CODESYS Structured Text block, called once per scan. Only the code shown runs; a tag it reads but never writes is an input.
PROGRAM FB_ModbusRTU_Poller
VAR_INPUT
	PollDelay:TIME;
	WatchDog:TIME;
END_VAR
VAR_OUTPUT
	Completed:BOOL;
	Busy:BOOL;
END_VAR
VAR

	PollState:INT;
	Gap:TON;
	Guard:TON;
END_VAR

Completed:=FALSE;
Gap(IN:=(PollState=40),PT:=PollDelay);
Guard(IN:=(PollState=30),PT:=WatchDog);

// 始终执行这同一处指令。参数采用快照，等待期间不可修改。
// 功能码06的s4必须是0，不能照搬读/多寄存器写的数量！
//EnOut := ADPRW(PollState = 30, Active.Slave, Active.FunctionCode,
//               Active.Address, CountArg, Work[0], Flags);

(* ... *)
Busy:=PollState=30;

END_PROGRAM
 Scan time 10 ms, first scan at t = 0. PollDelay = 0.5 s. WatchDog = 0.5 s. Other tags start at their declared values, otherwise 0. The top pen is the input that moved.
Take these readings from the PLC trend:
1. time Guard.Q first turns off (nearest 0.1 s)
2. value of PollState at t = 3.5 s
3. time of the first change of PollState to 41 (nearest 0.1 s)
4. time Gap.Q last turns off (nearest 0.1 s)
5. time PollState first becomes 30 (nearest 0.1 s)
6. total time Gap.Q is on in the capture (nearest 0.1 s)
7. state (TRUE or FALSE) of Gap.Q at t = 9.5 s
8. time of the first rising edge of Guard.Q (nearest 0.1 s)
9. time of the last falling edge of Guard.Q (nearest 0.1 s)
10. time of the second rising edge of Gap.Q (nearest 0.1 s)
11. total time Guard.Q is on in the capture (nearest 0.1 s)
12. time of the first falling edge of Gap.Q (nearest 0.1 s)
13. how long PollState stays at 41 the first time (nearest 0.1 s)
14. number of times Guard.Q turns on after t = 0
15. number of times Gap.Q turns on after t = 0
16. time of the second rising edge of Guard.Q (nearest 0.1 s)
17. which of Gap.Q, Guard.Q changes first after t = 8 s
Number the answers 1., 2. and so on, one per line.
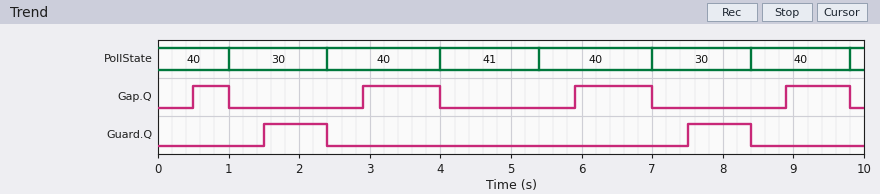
1. 2.4 s
2. 40
3. 4.0 s
4. 9.8 s
5. 1.0 s
6. 3.6 s
7. TRUE
8. 1.5 s
9. 8.4 s
10. 2.9 s
11. 1.8 s
12. 1.0 s
13. 1.4 s
14. 2
15. 4
16. 7.5 s
17. Guard.Q
